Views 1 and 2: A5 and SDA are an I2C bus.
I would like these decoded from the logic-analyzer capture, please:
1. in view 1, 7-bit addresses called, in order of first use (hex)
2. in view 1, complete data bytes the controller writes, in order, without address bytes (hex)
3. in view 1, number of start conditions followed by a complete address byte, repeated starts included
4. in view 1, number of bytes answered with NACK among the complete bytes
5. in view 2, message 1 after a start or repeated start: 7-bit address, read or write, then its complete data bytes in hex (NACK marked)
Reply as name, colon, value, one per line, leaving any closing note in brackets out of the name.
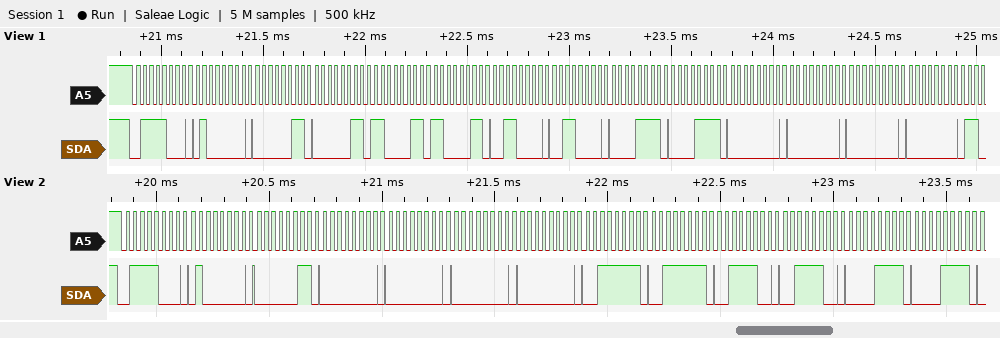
in view 1, 7-bit addresses called, in order of first use: 0x3C
in view 1, complete data bytes the controller writes, in order, without address bytes: 40 03 03 C3 C3 30 30 0F 0F 00 00 00 00
in view 1, number of start conditions followed by a complete address byte, repeated starts included: 1
in view 1, number of bytes answered with NACK among the complete bytes: 0
in view 2, message 1 after a start or repeated start: 7-bit address, read or write, then its complete data bytes in hex: 0x3C write: 40 03 00 00 00 00 3F 3F 3C 3C 0F 0F
